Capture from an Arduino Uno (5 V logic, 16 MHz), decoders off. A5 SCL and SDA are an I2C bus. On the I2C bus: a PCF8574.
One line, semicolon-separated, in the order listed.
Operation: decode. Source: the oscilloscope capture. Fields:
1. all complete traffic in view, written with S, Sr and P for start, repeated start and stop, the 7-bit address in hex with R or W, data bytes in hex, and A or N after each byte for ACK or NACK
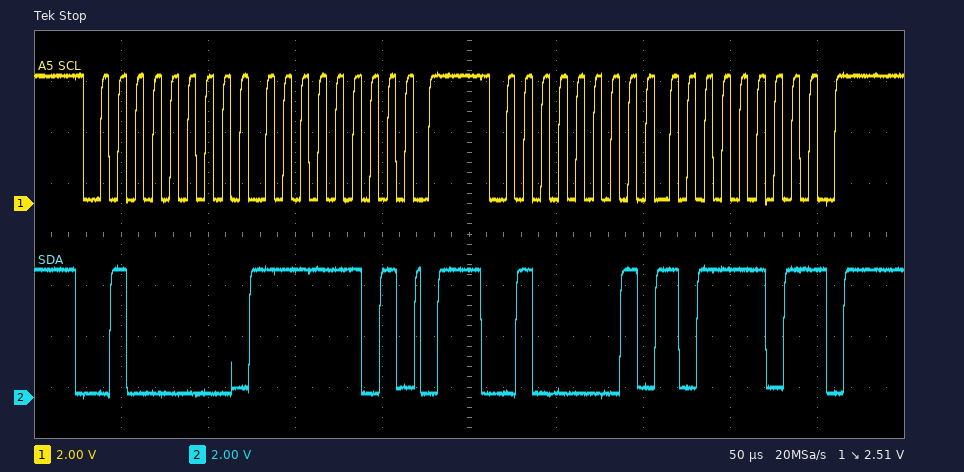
S 20W A FD A P S 20R A BD N P
